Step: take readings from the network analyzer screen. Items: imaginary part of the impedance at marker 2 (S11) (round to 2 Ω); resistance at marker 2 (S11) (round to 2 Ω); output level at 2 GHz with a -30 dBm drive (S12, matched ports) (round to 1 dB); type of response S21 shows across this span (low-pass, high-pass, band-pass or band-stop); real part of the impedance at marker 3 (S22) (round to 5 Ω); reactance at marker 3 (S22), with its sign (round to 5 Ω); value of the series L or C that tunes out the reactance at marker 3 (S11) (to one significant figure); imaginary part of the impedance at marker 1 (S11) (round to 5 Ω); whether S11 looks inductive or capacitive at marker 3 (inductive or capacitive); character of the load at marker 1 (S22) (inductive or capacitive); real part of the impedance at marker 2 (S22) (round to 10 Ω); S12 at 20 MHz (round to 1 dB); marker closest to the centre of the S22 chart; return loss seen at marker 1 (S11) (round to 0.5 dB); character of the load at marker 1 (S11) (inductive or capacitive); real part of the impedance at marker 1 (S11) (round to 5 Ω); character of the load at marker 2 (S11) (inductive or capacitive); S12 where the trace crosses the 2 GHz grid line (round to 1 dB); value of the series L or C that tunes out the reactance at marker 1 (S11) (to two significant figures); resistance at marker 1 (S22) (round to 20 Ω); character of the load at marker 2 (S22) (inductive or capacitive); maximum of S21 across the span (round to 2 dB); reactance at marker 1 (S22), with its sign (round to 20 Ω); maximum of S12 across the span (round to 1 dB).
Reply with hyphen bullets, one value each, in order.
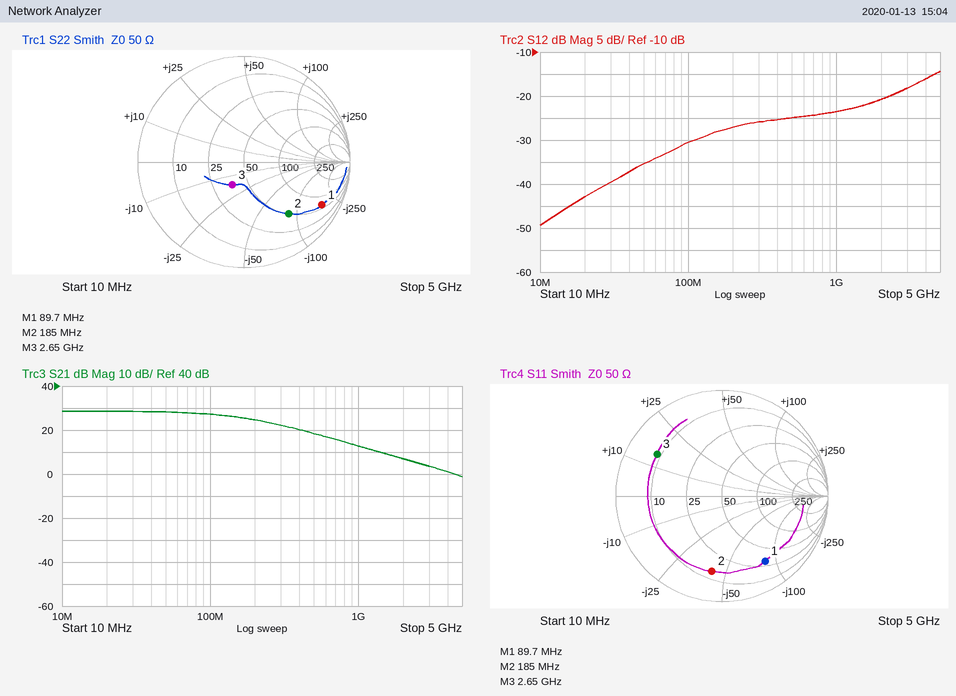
- -42 Ω
- 14 Ω
- -51 dBm
- low-pass
- 35 Ω
- -15 Ω
- 4 pF
- -85 Ω
- inductive
- capacitive
- 50 Ω
- -43 dB
- marker 3
- 2.5 dB
- capacitive
- 30 Ω
- capacitive
- -21 dB
- 150 nH
- 60 Ω
- capacitive
- 28 dB
- -180 Ω
- -14 dB
